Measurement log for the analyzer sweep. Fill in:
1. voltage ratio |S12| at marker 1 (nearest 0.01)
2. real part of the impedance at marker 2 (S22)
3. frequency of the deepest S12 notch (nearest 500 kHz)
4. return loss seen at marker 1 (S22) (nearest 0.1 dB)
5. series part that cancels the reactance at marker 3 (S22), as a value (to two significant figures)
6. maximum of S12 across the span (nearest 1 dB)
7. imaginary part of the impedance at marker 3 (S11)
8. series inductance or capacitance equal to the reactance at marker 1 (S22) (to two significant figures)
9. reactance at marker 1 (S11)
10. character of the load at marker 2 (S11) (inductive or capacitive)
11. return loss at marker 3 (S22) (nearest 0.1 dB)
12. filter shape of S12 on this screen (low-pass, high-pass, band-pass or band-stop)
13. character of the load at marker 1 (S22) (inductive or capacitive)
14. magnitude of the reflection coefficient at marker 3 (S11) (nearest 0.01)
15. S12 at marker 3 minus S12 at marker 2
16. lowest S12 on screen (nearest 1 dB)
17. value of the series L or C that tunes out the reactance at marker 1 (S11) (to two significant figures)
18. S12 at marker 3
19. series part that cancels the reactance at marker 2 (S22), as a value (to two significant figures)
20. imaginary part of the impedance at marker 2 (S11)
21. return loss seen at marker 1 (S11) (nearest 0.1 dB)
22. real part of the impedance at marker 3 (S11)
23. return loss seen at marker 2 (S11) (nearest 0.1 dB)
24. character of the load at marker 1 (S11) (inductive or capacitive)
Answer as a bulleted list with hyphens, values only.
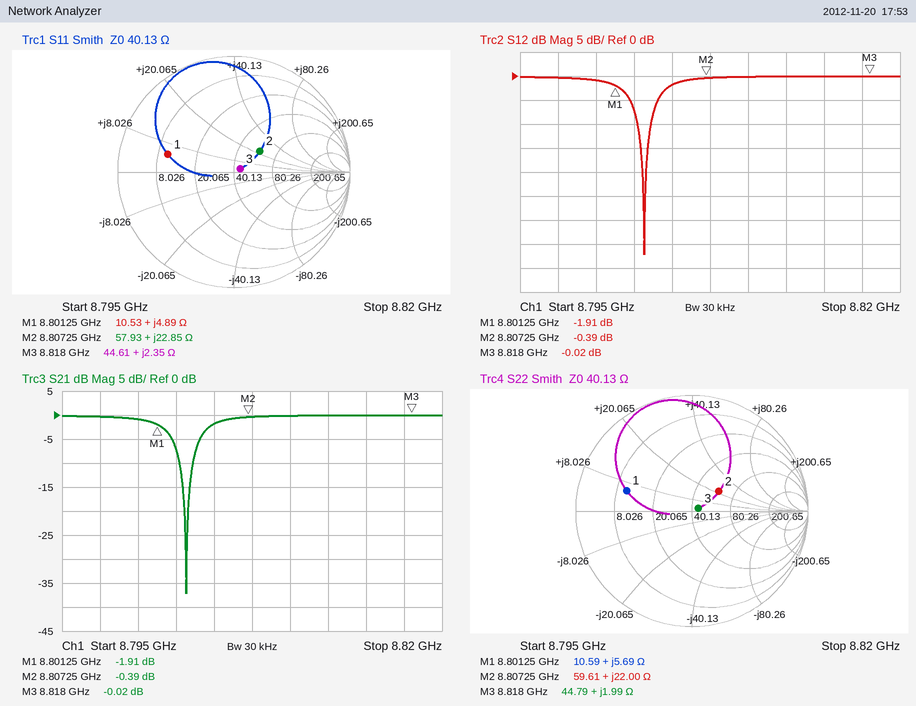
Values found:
- 0.80
- 59.61 Ω
- 8.8030 GHz
- 4.6 dB
- 9.1 pF
- 0 dB
- +2.35 Ω
- 100 pH
- +4.89 Ω
- inductive
- 24.5 dB
- band-stop
- inductive
- 0.06
- 0.37 dB
- -37 dB
- 3.7 pF
- -0.02 dB
- 820 fF
- +22.85 Ω
- 4.6 dB
- 44.61 Ω
- 10.8 dB
- inductive
